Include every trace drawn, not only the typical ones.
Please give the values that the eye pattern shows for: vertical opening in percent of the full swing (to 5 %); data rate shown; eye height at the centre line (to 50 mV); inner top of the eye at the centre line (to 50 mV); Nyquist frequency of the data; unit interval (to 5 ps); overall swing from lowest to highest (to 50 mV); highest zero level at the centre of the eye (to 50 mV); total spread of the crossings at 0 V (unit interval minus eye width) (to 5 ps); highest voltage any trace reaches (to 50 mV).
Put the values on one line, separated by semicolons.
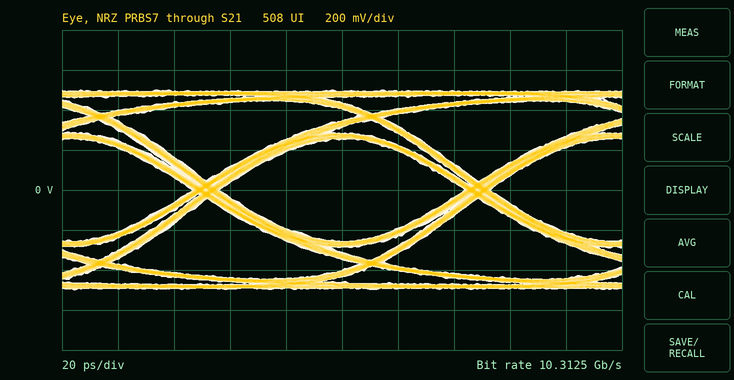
50 %; 10.3125 Gb/s; 500 mV; 250 mV; 5.15625 GHz; 95 ps; 1.00 V; -250 mV; 10 ps; 500 mV
